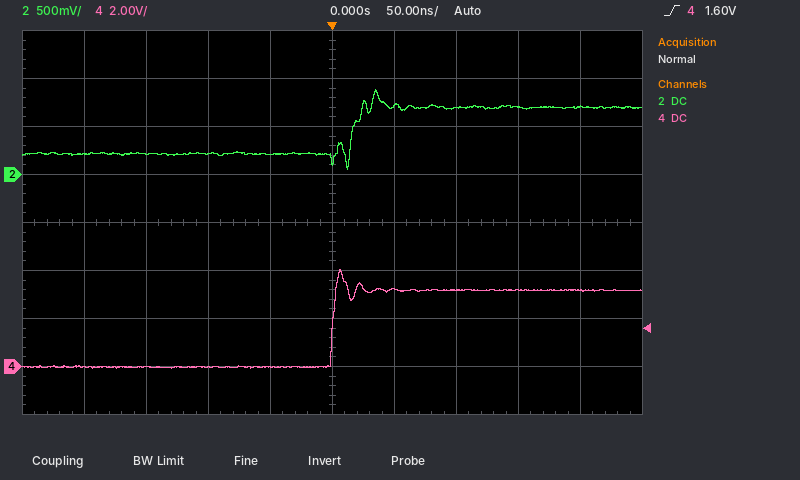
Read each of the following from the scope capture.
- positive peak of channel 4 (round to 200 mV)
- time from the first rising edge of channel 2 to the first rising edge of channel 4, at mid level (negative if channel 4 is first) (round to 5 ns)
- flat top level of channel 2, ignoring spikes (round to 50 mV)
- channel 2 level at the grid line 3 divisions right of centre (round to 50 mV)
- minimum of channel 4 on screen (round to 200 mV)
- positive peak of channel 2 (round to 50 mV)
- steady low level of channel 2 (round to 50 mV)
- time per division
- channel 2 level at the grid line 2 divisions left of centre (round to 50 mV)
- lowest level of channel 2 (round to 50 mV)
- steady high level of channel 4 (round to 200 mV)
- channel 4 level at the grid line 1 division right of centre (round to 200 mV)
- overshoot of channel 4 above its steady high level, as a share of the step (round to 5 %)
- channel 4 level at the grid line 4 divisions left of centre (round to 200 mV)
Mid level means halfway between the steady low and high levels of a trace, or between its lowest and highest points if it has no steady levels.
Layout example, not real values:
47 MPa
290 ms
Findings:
4.0 V
-15 ns
700 mV
700 mV
0.0 V
900 mV
200 mV
50 ns
200 mV
50 mV
3.2 V
3.2 V
25 %
0.0 V
